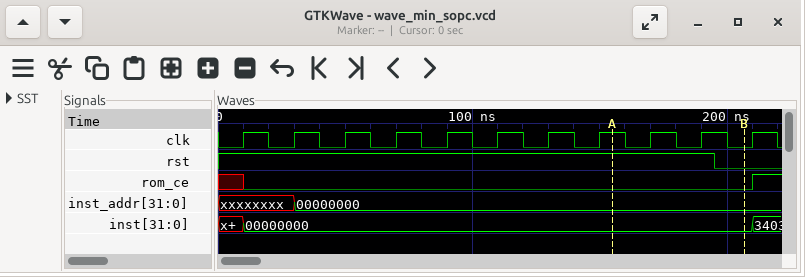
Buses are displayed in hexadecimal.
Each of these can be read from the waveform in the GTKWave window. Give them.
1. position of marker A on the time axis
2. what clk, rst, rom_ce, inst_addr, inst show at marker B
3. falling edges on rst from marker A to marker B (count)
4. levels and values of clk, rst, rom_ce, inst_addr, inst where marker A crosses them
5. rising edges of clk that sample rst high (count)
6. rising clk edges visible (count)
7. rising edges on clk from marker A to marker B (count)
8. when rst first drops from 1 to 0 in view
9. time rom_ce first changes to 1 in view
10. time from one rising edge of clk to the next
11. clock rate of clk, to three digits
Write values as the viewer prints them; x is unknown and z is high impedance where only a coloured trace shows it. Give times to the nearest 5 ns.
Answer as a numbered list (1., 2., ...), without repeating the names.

1. 155 ns
2. clk=0, rst=0, rom_ce=0, inst_addr=00000000, inst=00000000
3. 1
4. clk=1, rst=1, rom_ce=0, inst_addr=00000000, inst=00000000
5. 10
6. 11
7. 2
8. 195 ns
9. 210 ns
10. 20 ns
11. 50.0 MHz
